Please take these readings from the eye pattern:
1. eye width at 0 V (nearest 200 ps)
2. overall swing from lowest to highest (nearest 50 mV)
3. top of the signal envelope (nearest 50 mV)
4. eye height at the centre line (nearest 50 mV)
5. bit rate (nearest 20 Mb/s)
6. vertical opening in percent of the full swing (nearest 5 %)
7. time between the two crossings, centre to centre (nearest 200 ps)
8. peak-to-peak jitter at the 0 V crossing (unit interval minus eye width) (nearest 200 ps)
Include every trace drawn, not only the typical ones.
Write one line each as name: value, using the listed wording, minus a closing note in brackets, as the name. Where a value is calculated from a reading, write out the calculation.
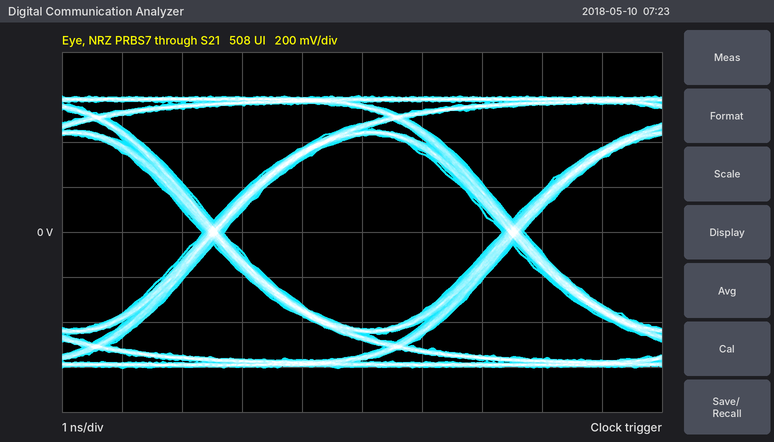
eye width at 0 V: 4.6 ns
overall swing from lowest to highest: 1.20 V
top of the signal envelope: 600 mV
eye height at the centre line: 850 mV
bit rate: 200 Mb/s
vertical opening in percent of the full swing: 850 mV / 1.20 V ≈ 70.8 %, so 70 % to the nearest 5 %
time between the two crossings, centre to centre: 5.0 ns
peak-to-peak jitter at the 0 V crossing (unit interval minus eye width): 400 ps
